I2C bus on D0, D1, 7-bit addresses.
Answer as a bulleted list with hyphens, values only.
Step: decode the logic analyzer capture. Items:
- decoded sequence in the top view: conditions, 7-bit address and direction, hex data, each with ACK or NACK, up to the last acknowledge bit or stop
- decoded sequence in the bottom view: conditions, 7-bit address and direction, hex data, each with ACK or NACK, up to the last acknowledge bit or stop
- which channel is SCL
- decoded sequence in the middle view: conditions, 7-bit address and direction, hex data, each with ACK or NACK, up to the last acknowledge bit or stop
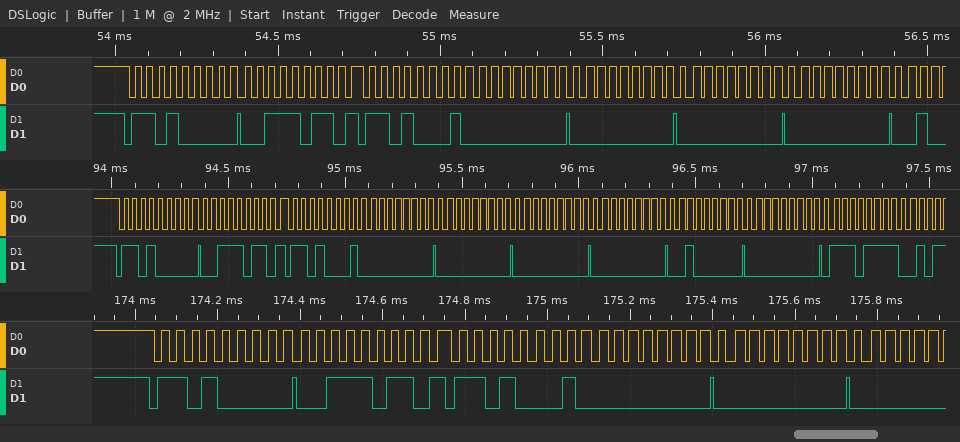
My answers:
- start, address 68 write ACK, 3B ACK, repeated start, address 68 read ACK, 00 ACK, 00 ACK, 00 ACK, 00 ACK
- start, address 68 write ACK, 3B ACK, repeated start, address 68 read ACK, 00 ACK, 00 ACK
- D0
- start, address 68 write ACK, 3B ACK, repeated start, address 68 read ACK, 00 ACK, 00 ACK, 00 ACK, 00 ACK, 40 ACK, 00 ACK, EF ACK
